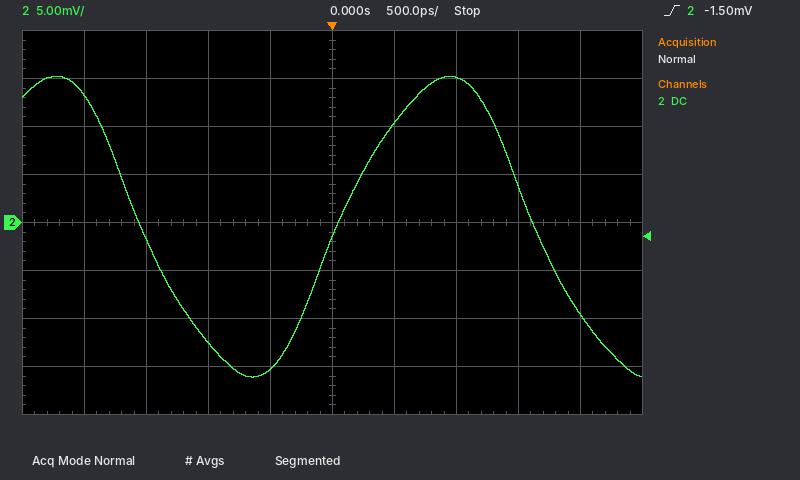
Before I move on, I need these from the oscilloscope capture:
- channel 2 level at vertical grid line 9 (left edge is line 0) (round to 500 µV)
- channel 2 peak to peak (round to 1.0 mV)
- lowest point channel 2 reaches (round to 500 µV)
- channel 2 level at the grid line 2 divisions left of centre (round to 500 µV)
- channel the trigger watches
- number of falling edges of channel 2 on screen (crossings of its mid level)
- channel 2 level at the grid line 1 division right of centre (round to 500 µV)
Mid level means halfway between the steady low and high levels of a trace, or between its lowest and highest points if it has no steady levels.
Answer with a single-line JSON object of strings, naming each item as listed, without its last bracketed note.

{"channel 2 level at vertical grid line 9 (left edge is line 0)": "-9.5 mV", "channel 2 peak to peak": "31.0 mV", "lowest point channel 2 reaches": "-16.0 mV", "channel 2 level at the grid line 2 divisions left of centre": "-12.5 mV", "channel the trigger watches": "channel 2", "number of falling edges of channel 2 on screen": "2", "channel 2 level at the grid line 1 division right of centre": "10.5 mV"}
